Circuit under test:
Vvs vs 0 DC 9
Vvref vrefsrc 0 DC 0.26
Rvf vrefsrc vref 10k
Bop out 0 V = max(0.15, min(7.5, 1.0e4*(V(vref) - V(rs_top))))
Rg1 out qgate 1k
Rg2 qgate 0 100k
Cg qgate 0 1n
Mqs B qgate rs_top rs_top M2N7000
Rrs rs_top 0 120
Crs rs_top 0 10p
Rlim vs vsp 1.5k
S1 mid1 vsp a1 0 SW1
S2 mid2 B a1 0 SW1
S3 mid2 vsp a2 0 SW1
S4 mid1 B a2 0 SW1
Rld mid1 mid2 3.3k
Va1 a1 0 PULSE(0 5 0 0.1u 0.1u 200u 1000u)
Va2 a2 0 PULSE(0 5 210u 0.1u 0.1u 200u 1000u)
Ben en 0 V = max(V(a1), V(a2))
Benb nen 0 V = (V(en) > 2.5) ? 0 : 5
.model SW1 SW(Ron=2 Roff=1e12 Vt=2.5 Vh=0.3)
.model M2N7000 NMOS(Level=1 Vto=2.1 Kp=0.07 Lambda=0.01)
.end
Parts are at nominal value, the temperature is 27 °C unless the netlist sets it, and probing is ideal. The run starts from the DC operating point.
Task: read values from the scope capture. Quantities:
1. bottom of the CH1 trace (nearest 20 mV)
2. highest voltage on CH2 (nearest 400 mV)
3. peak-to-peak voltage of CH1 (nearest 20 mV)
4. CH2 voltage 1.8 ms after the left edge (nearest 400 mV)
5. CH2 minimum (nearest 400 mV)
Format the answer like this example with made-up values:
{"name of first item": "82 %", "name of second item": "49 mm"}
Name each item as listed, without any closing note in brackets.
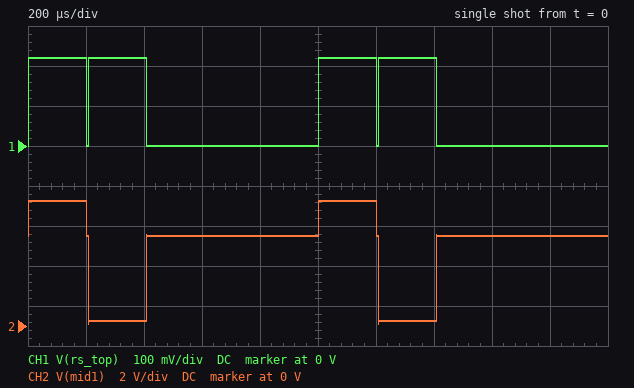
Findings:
{"bottom of the CH1 trace": "0 V", "highest voltage on CH2": "6.4 V", "peak-to-peak voltage of CH1": "220 mV", "CH2 voltage 1.8 ms after the left edge": "4.4 V", "CH2 minimum": "0 V"}
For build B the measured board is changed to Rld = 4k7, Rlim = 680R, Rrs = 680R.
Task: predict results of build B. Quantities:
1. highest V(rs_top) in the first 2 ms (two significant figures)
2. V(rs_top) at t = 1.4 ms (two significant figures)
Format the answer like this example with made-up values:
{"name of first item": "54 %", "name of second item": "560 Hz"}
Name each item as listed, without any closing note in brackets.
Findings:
{"highest V(rs_top) in the first 2 ms": "1.0 V", "V(rs_top) at t = 1.4 ms": "260 mV"}
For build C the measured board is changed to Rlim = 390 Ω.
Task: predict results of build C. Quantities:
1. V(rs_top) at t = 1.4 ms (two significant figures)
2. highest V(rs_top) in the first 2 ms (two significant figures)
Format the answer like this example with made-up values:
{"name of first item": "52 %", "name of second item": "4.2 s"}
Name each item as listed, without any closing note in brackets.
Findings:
{"V(rs_top) at t = 1.4 ms": "260 mV", "highest V(rs_top) in the first 2 ms": "280 mV"}
